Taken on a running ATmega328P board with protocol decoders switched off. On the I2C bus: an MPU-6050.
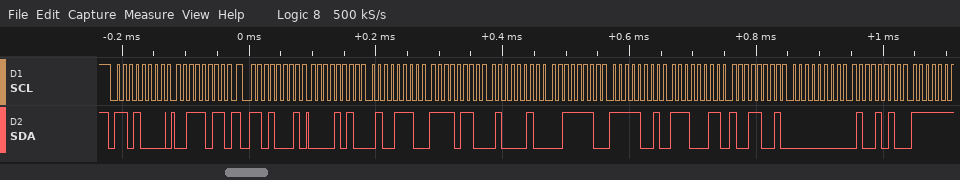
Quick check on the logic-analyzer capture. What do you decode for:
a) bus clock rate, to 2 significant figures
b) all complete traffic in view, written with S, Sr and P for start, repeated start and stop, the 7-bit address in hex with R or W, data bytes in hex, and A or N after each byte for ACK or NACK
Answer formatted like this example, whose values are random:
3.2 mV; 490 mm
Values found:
100 kHz; S 68W A 3B A Sr 68R A 0A A 4E A F6 A 42 A 3E A F9 A E3 A 99 A 00 A 4A A
